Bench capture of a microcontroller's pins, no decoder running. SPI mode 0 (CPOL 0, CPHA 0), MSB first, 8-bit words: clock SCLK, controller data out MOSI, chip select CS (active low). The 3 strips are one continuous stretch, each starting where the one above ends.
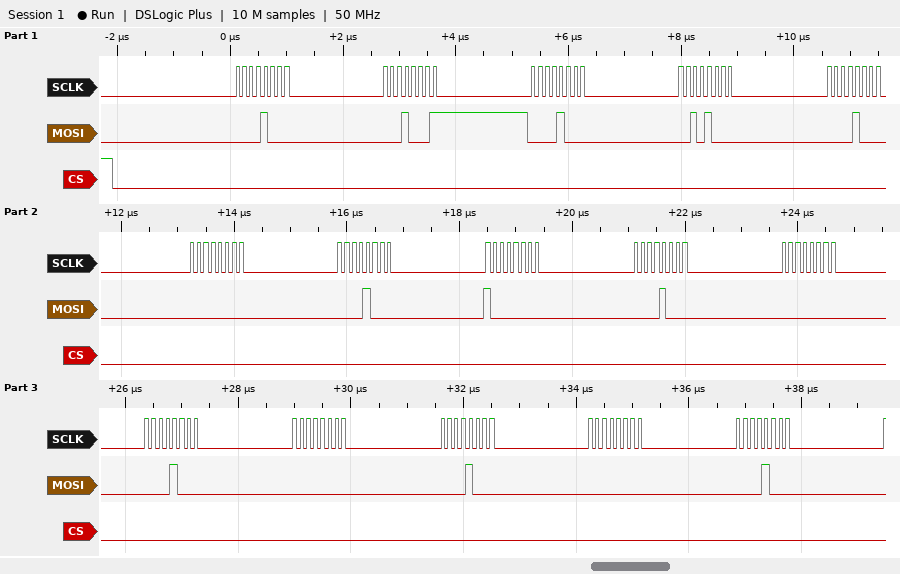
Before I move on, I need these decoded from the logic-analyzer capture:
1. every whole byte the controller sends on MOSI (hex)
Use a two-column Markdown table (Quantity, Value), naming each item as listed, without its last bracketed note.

| Quantity | Value |
|---|---|
| every whole byte the controller sends on MOSI | 08 11 08 28 08 00 08 80 08 00 08 00 08 00 08 |
